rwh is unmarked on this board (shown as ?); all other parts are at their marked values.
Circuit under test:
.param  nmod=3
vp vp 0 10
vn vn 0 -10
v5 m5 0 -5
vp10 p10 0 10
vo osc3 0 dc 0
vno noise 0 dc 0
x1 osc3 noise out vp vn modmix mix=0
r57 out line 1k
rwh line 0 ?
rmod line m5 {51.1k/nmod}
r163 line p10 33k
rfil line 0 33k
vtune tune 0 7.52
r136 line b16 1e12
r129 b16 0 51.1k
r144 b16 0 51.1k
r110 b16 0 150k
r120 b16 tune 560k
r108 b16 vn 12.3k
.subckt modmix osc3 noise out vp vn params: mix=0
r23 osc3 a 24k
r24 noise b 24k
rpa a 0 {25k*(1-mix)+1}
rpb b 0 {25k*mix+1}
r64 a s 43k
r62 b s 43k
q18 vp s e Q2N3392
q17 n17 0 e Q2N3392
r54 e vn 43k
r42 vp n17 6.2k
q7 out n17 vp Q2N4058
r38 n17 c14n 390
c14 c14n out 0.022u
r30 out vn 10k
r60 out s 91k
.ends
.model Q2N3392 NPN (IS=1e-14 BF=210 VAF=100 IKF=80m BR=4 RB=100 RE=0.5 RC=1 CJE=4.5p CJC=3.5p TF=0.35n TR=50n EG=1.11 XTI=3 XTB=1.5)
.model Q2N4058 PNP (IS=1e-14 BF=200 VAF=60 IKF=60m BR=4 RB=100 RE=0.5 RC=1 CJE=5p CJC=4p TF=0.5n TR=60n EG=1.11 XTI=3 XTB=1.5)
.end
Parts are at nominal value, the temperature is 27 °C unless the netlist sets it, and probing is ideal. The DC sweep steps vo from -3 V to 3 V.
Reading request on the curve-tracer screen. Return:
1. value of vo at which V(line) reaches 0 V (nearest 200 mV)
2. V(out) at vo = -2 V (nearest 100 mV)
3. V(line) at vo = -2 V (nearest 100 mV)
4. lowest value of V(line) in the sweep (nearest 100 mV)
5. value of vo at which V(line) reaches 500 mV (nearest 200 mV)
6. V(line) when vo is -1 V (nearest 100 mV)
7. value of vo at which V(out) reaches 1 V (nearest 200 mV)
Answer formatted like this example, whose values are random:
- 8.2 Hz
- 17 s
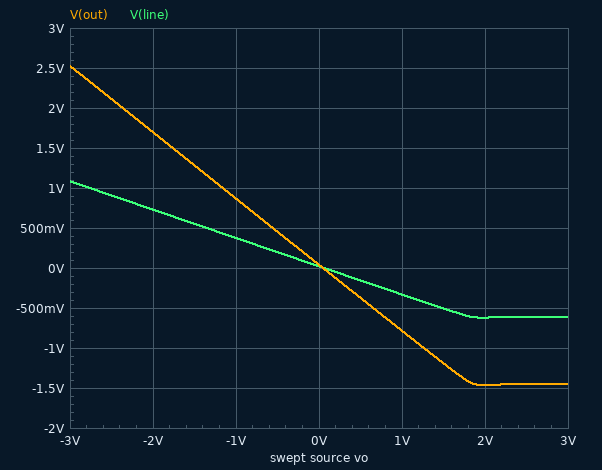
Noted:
- 0 V
- 1.7 V
- 700 mV
- -600 mV
- -1.4 V
- 400 mV
- -1.2 V
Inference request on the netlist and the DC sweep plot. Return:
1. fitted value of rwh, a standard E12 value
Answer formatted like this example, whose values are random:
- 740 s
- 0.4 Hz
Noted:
- 820 Ω
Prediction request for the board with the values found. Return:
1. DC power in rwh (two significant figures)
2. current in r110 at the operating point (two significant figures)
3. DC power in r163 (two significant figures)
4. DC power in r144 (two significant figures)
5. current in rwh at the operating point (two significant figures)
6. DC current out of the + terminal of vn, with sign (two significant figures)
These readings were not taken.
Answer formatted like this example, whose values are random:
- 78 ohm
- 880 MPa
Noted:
- 540 nW
- 41 µA
- 3.0 mW
- 750 µW
- 26 µA
- -1.5 mA
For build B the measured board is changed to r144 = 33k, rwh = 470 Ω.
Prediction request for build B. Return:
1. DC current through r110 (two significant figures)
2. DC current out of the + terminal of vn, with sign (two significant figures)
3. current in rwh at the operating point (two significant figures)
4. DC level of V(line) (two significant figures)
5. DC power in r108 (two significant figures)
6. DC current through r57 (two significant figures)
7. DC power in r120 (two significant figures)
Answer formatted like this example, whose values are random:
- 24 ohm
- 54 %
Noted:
- 38 µA
- -1.6 mA
- 32 µA
- 15 mV
- 1.5 mW
- 24 µA
- 310 µW
